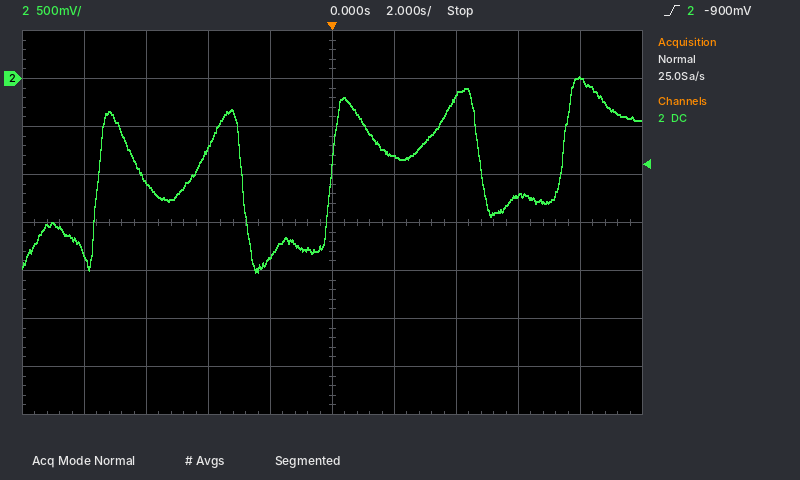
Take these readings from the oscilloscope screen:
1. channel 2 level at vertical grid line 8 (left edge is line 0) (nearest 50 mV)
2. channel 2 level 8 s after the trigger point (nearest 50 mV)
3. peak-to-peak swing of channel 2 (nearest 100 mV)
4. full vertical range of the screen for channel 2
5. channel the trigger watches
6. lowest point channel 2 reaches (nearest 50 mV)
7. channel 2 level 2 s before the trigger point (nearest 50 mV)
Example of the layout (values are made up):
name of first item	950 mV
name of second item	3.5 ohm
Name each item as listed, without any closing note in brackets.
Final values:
channel 2 level at vertical grid line 8 (left edge is line 0)	-1.20 V
channel 2 level 8 s after the trigger point	0 mV
peak-to-peak swing of channel 2	2.00 V
full vertical range of the screen for channel 2	4 V
channel the trigger watches	channel 2
lowest point channel 2 reaches	-2.00 V
channel 2 level 2 s before the trigger point	-1.85 V
